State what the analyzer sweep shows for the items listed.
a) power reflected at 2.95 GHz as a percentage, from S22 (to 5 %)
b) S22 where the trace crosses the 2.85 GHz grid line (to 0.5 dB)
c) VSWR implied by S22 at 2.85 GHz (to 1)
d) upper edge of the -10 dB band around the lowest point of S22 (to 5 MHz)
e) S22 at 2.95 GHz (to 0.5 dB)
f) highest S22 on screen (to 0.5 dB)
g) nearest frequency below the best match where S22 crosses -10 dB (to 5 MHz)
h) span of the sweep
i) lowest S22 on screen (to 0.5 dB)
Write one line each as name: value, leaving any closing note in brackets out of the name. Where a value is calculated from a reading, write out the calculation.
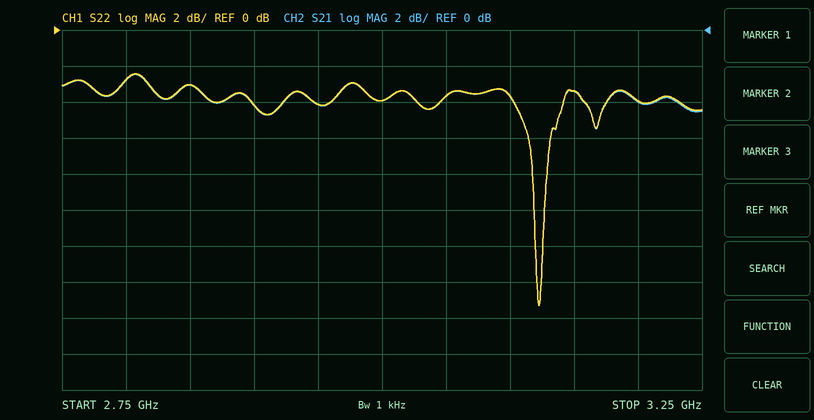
power reflected at 2.95 GHz as a percentage, from S22: 10^(-4/10) ≈ 40 %
S22 where the trace crosses the 2.85 GHz grid line: -3.0 dB
VSWR implied by S22 at 2.85 GHz: |Γ| = 10^(-3/20) = 0.7079; VSWR = (1 + 0.7079)/(1 − 0.7079) ≈ 6
upper edge of the -10 dB band around the lowest point of S22: 3.125 GHz
S22 at 2.95 GHz: -4.0 dB
highest S22 on screen: -2.5 dB
nearest frequency below the best match where S22 crosses -10 dB: 3.120 GHz
span of the sweep: 500 MHz
lowest S22 on screen: -15.5 dB
